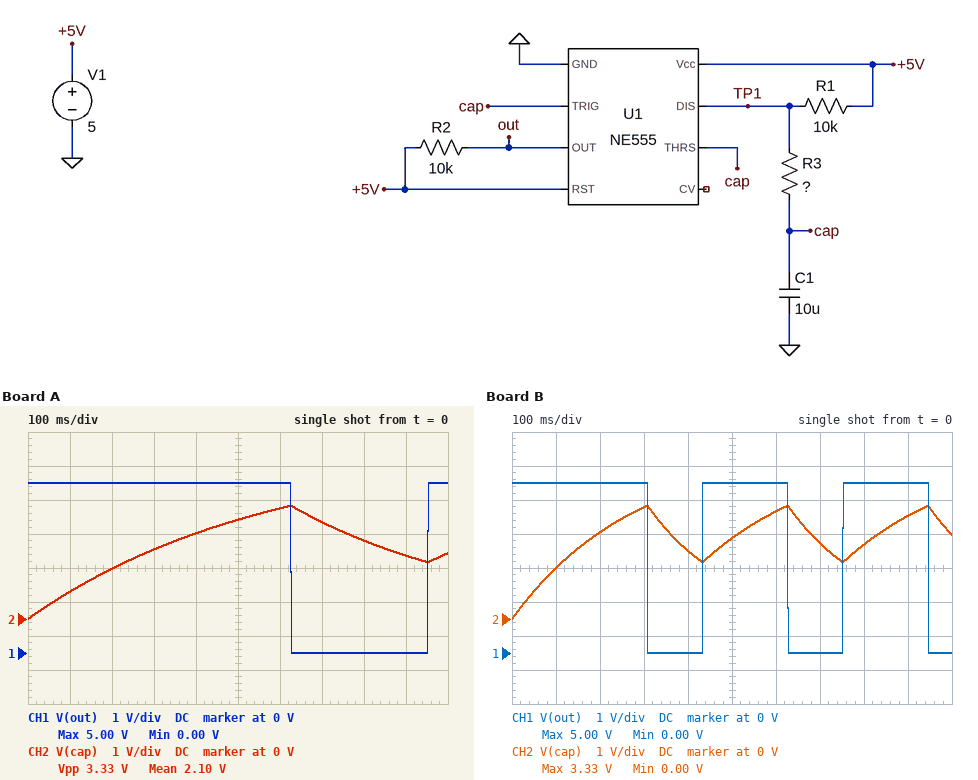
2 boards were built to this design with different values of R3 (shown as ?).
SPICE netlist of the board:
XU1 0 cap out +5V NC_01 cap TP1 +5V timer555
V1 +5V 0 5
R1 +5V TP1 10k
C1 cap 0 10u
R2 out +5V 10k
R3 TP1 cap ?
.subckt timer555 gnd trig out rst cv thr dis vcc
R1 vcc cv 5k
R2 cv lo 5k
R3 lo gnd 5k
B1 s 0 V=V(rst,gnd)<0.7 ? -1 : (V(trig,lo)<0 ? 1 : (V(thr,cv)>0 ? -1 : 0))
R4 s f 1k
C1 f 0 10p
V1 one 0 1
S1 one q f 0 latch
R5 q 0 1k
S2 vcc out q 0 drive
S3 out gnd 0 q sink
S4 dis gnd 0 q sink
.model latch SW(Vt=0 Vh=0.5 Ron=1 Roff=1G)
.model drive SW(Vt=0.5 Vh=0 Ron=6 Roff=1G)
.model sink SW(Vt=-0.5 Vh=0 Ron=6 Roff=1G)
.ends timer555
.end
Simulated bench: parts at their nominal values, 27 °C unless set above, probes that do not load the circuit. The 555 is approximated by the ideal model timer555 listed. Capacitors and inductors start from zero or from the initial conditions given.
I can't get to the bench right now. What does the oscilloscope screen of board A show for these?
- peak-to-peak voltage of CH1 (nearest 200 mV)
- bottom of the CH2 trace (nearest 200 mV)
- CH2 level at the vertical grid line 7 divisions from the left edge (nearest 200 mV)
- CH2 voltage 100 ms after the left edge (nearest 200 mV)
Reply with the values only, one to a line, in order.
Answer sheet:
5.0 V
0 V
2.8 V
800 mV
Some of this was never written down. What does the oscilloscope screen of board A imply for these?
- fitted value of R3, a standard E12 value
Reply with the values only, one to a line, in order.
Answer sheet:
47 kΩ
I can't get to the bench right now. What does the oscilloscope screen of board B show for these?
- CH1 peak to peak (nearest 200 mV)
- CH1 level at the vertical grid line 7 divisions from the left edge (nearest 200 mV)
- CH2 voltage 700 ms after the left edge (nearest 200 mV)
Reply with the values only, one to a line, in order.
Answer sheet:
5.0 V
0 V
2.2 V
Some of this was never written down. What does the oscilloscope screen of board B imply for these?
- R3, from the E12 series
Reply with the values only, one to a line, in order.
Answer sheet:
18 kΩ
